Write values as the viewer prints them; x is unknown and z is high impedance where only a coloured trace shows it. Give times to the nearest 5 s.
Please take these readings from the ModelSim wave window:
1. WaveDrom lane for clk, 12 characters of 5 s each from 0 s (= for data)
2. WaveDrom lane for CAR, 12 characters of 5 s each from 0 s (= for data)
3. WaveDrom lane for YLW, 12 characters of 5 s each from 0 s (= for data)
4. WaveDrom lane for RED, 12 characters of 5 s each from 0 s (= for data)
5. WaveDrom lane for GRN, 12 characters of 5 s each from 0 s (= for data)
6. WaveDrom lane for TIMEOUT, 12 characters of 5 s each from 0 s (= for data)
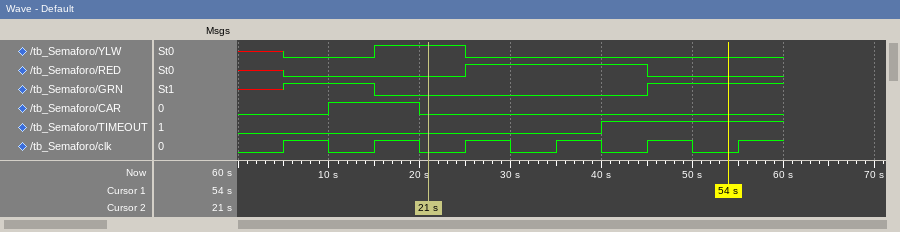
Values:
{name: 'clk', wave: '010101010101'}
{name: 'CAR', wave: '0.1.0.......'}
{name: 'YLW', wave: 'x0.1.0......'}
{name: 'RED', wave: 'x0...1...0..'}
{name: 'GRN', wave: 'x1.0.....1..'}
{name: 'TIMEOUT', wave: '0.......1...'}
